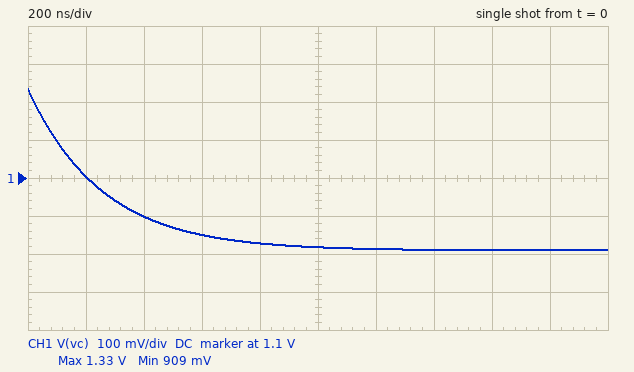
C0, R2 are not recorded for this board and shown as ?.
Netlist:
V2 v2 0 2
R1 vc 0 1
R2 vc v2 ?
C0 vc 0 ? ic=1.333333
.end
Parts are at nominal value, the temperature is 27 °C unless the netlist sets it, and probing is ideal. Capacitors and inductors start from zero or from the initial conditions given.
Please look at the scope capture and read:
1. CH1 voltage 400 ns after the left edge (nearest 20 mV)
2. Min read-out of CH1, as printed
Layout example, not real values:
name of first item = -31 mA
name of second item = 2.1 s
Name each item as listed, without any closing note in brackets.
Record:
CH1 voltage 400 ns after the left edge = 1.00 V
Min read-out of CH1, as printed = 909 mV
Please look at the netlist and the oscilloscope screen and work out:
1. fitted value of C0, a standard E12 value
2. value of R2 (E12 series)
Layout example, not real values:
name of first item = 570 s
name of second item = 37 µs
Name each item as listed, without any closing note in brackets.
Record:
fitted value of C0, a standard E12 value = 470 nF
value of R2 = 1.2 Ω
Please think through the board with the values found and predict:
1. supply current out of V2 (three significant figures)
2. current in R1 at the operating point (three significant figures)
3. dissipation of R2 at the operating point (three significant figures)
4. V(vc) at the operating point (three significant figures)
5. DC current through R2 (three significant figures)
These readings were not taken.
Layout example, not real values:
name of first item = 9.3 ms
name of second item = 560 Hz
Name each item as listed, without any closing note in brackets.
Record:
supply current out of V2 = 909 mA
current in R1 at the operating point = 909 mA
dissipation of R2 at the operating point = 992 mW
V(vc) at the operating point = 909 mV
DC current through R2 = 909 mA
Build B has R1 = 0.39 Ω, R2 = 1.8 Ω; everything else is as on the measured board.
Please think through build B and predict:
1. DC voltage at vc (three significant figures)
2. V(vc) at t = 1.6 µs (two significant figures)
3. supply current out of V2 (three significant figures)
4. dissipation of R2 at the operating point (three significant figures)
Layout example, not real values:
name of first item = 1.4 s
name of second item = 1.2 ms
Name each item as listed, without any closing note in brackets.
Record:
DC voltage at vc = 356 mV
V(vc) at t = 1.6 µs = 360 mV
supply current out of V2 = 913 mA
dissipation of R2 at the operating point = 1.50 W
